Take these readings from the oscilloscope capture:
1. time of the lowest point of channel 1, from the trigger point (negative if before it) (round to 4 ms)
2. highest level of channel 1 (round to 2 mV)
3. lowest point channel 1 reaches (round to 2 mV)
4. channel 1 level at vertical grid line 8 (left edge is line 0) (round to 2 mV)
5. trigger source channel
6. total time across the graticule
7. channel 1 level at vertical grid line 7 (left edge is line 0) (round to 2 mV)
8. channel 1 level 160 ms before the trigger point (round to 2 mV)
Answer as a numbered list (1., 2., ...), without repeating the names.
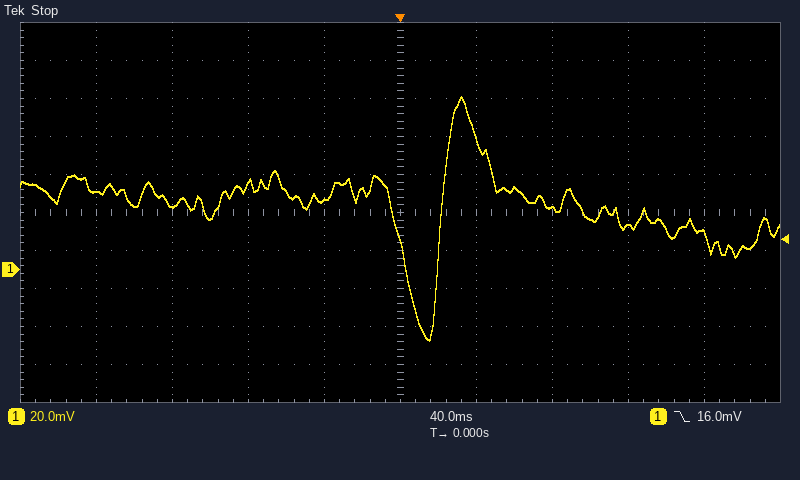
1. +16 ms
2. 92 mV
3. -38 mV
4. 22 mV
5. channel 1
6. 400 ms
7. 32 mV
8. 40 mV
